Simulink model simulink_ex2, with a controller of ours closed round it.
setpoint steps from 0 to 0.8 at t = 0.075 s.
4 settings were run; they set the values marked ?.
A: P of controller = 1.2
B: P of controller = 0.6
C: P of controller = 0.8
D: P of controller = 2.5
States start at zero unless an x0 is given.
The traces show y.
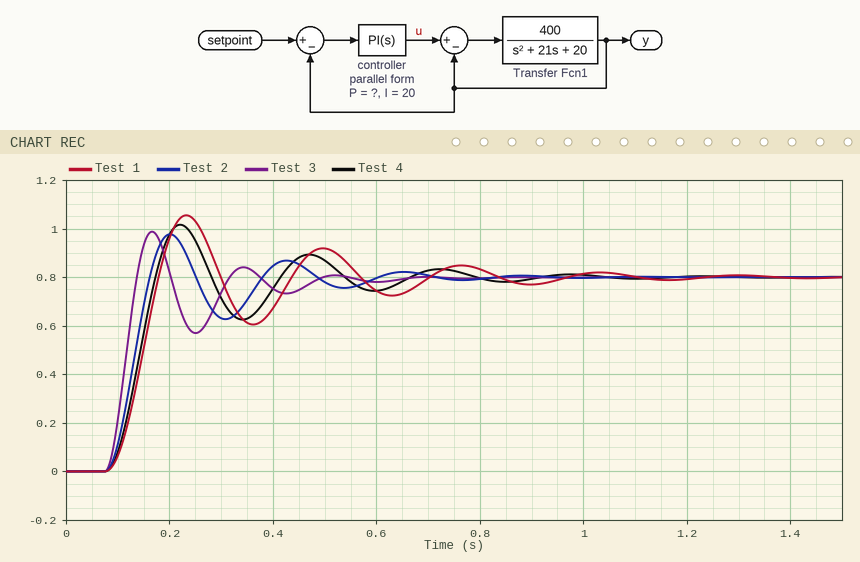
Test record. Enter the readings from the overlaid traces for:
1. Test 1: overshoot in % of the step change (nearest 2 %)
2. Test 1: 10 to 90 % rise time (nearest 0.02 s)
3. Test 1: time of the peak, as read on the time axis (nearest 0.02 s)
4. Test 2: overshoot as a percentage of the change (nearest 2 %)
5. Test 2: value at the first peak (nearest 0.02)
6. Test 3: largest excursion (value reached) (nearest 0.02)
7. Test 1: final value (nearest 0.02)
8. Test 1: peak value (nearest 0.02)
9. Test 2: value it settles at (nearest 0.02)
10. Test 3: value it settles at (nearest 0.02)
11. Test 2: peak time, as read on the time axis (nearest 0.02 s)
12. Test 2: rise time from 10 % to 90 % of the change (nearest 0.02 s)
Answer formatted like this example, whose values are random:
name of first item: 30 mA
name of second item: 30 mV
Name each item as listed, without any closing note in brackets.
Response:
Test 1: overshoot in % of the step change: 32 %
Test 1: 10 to 90 % rise time: 0.06 s
Test 1: time of the peak, as read on the time axis: 0.24 s
Test 2: overshoot as a percentage of the change: 22 %
Test 2: value at the first peak: 0.98
Test 3: largest excursion (value reached): 0.98
Test 1: final value: 0.80
Test 1: peak value: 1.06
Test 2: value it settles at: 0.80
Test 3: value it settles at: 0.80
Test 2: peak time, as read on the time axis: 0.20 s
Test 2: rise time from 10 % to 90 % of the change: 0.06 s
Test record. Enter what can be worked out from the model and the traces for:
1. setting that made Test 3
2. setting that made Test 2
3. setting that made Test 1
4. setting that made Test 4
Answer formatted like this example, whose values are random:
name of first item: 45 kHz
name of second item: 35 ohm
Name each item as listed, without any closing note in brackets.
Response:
setting that made Test 3: D
setting that made Test 2: A
setting that made Test 1: B
setting that made Test 4: C
